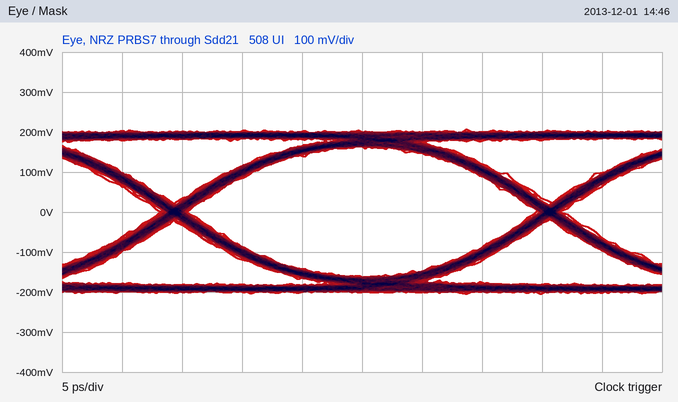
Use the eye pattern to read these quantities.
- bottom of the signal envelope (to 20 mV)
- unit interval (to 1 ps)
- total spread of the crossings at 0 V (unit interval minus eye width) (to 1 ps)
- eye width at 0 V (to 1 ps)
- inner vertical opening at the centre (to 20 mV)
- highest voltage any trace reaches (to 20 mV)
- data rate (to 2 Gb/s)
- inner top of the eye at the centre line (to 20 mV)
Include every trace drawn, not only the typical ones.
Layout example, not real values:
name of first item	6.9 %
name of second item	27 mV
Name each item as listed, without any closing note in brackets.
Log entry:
bottom of the signal envelope	-200 mV
unit interval	31 ps
total spread of the crossings at 0 V (unit interval minus eye width)	2 ps
eye width at 0 V	29 ps
inner vertical opening at the centre	320 mV
highest voltage any trace reaches	200 mV
data rate	32 Gb/s
inner top of the eye at the centre line	160 mV
